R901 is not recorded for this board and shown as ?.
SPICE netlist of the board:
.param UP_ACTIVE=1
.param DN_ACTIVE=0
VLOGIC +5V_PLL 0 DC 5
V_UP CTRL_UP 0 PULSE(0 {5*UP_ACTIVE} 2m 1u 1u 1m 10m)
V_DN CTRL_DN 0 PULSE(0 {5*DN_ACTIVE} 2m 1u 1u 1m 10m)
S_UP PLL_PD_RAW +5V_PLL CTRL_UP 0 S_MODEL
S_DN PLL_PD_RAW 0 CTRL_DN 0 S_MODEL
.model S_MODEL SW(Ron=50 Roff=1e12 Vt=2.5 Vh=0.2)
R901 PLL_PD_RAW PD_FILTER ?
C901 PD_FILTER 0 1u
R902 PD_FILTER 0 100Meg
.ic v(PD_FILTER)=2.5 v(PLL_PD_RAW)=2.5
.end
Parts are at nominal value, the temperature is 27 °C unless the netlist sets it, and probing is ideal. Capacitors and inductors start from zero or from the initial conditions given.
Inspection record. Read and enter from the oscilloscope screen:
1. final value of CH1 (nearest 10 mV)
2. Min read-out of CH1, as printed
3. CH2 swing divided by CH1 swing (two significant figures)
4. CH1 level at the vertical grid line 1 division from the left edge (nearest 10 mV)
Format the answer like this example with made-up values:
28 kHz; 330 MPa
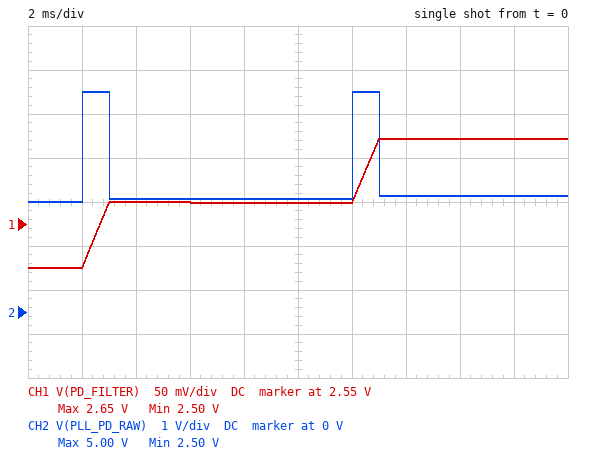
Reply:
2.65 V; 2.50 V; 17; 2.50 V
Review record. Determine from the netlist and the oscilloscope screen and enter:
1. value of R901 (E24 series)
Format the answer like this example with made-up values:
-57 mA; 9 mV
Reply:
33 kΩ
